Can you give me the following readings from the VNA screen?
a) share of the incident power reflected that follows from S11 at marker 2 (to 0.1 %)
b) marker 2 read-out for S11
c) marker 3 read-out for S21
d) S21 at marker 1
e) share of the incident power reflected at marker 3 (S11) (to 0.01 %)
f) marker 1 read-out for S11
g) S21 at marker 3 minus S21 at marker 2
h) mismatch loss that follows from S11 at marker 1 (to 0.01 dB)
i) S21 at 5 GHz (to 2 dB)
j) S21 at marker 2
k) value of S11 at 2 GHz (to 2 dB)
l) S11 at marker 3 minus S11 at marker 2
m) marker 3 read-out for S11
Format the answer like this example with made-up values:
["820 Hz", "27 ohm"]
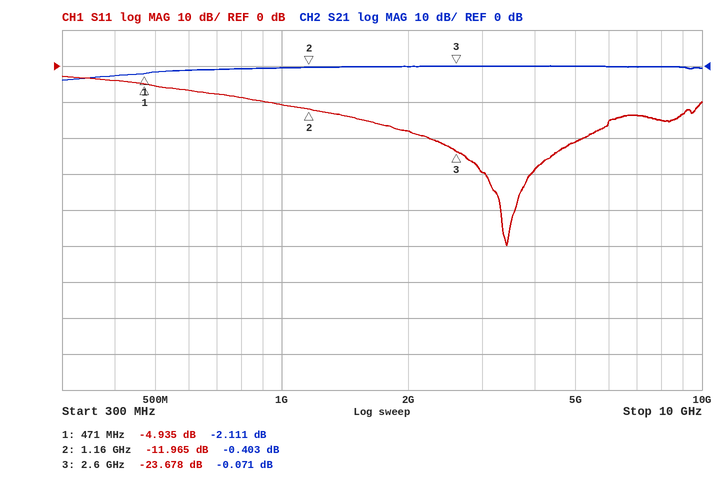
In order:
["6.4 %", "-11.965 dB", "-0.071 dB", "-2.111 dB", "0.43 %", "-4.935 dB", "0.332 dB", "1.68 dB", "0 dB", "-0.403 dB", "-18 dB", "-11.713 dB", "-23.678 dB"]
